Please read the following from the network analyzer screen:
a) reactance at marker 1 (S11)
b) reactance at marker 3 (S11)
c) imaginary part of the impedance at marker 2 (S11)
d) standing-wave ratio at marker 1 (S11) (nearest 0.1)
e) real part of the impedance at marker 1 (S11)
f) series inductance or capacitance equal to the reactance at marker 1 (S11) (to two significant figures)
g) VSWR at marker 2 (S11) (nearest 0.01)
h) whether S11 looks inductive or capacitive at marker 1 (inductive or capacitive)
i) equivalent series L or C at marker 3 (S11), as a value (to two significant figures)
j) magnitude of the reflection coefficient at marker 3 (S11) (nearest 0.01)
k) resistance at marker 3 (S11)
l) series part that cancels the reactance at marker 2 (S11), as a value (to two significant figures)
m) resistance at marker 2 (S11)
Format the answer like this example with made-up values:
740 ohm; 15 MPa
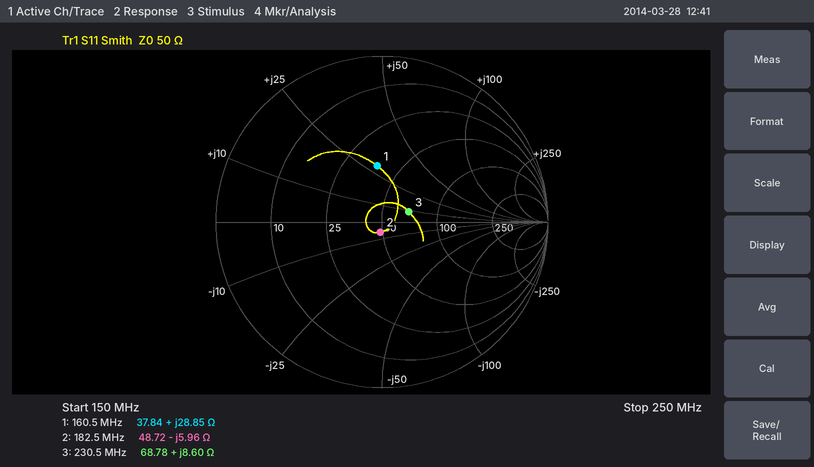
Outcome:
+28.85 Ω; +8.60 Ω; -5.96 Ω; 2.0; 37.84 Ω; 29 nH; 1.13; inductive; 5.9 nH; 0.17; 68.78 Ω; 5.2 nH; 48.72 Ω
